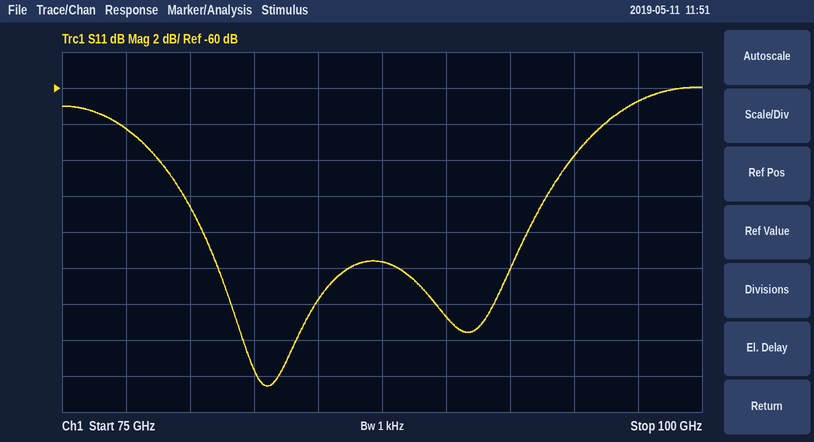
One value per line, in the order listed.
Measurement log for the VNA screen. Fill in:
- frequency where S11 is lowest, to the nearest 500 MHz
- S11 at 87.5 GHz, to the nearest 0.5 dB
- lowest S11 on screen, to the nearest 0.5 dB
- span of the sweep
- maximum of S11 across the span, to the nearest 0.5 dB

83.0 GHz
-69.5 dB
-76.5 dB
25 GHz
-60.0 dB
